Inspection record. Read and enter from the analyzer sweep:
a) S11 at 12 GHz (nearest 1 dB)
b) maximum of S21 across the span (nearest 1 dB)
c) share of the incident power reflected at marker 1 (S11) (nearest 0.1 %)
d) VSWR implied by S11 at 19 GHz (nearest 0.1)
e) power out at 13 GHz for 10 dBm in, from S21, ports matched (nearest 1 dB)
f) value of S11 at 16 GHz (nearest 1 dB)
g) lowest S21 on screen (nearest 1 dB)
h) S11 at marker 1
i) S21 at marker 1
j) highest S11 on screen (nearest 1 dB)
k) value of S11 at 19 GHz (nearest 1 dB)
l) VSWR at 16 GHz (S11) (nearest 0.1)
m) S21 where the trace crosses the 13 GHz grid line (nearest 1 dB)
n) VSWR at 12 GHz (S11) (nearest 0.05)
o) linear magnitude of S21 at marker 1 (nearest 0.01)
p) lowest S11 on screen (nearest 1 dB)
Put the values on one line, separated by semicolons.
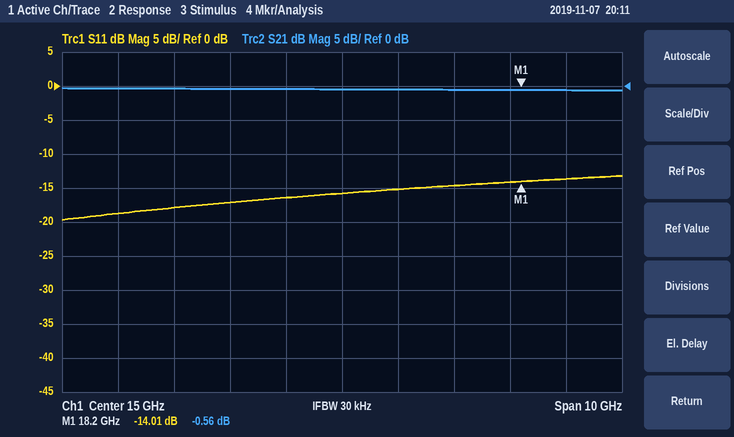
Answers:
-18 dB; 0 dB; 4.0 %; 1.5; 10 dBm; -15 dB; -1 dB; -14.01 dB; -0.56 dB; -13 dB; -14 dB; 1.4; 0 dB; 1.30; 0.94; -20 dB
